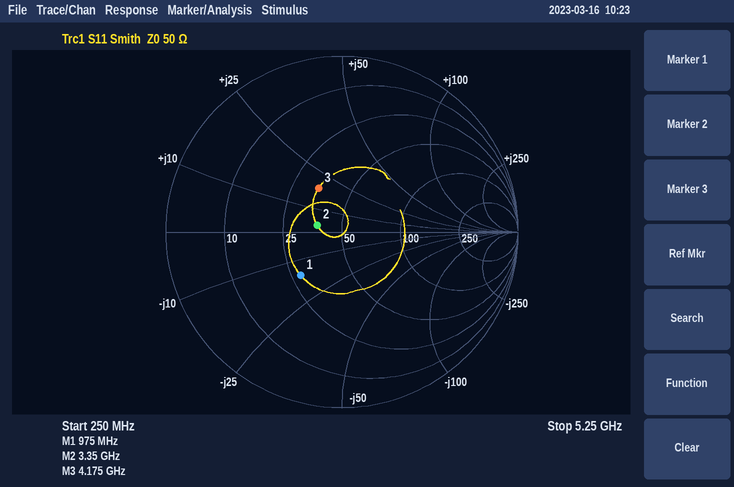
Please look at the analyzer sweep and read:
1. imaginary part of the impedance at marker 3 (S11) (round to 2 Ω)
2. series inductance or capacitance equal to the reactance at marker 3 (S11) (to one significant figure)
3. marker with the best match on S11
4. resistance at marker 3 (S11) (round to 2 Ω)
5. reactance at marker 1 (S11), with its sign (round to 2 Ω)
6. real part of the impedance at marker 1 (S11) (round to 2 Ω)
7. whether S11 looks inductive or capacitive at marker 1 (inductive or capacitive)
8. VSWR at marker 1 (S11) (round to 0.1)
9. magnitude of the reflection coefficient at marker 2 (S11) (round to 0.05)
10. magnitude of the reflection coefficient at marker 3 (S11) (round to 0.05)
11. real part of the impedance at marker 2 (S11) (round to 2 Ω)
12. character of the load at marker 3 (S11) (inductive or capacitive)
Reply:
+18 Ω
700 pH
marker 2
34 Ω
-16 Ω
28 Ω
capacitive
2.0
0.15
0.30
38 Ω
inductive
